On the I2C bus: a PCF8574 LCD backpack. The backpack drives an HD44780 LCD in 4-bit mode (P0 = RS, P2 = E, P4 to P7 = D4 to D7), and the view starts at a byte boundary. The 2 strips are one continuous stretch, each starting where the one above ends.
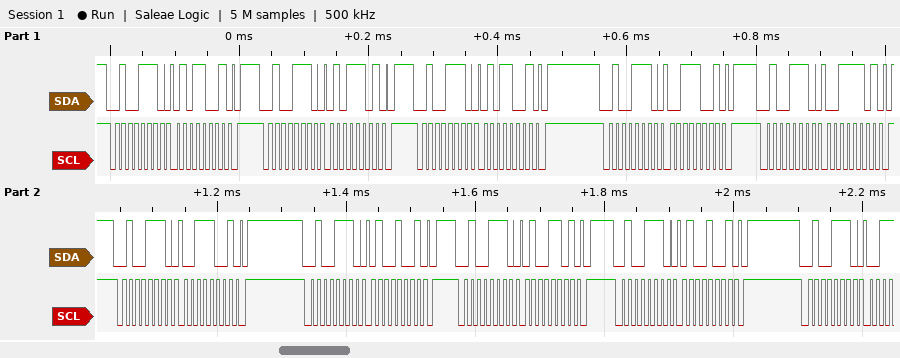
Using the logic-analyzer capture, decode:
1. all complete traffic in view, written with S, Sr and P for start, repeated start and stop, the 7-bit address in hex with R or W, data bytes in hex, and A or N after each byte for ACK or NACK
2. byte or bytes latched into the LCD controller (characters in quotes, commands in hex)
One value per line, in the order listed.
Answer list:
S 27W A 59 A P S 27W A 5D A P S 27W A 59 A P S 27W A 39 A P S 27W A 3D A P S 27W A 39 A P S 27W A 49 A P S 27W A 4D A P S 27W A 49 A P S 27W A
'S'
